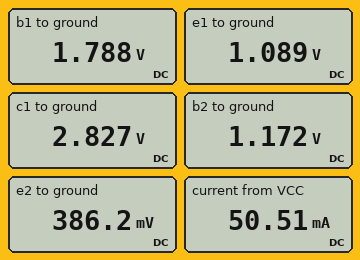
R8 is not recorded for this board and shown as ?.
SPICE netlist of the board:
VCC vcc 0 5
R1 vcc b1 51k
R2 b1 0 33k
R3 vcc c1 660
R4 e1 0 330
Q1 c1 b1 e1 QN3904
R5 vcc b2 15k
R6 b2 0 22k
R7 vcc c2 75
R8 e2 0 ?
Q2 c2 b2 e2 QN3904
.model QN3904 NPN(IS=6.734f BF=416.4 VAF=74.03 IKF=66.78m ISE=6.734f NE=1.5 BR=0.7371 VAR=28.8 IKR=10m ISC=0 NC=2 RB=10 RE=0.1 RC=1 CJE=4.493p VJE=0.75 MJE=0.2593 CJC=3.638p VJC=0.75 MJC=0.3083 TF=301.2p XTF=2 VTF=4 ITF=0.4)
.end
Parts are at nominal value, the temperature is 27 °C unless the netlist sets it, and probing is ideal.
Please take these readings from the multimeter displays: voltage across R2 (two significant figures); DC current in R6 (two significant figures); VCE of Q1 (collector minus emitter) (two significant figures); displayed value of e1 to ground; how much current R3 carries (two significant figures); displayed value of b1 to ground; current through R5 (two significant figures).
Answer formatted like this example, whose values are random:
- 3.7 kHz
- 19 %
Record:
- 1.8 V
- 53 µA
- 1.7 V
- 1.089 V
- 3.3 mA
- 1.788 V
- 260 µA
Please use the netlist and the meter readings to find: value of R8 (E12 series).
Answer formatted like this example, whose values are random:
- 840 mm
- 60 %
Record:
- 8.2 Ω
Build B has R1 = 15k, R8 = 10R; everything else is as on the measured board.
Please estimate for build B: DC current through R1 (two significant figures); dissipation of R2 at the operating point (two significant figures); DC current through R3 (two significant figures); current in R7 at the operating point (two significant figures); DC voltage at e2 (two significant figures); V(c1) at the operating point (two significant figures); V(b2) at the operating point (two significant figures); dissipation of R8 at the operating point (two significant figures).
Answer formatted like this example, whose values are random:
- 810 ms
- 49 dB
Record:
- 180 µA
- 170 µW
- 4.9 mA
- 46 mA
- 460 mV
- 1.8 V
- 1.2 V
- 21 mW
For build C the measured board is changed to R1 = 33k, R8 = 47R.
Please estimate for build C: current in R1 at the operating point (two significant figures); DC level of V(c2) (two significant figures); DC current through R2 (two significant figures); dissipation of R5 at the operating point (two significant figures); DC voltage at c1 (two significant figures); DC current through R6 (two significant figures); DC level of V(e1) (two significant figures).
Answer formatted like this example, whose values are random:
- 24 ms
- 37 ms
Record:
- 82 µA
- 2.9 V
- 69 µA
- 570 µW
- 1.9 V
- 95 µA
- 1.6 V
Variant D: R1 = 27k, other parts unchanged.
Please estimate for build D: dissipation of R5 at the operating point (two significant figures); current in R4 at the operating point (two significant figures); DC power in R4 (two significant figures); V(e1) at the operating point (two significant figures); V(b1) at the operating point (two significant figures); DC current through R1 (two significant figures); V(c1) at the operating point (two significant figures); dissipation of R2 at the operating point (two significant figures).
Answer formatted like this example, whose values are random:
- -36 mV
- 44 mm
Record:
- 980 µW
- 4.9 mA
- 7.9 mW
- 1.6 V
- 2.3 V
- 99 µA
- 1.8 V
- 160 µW
